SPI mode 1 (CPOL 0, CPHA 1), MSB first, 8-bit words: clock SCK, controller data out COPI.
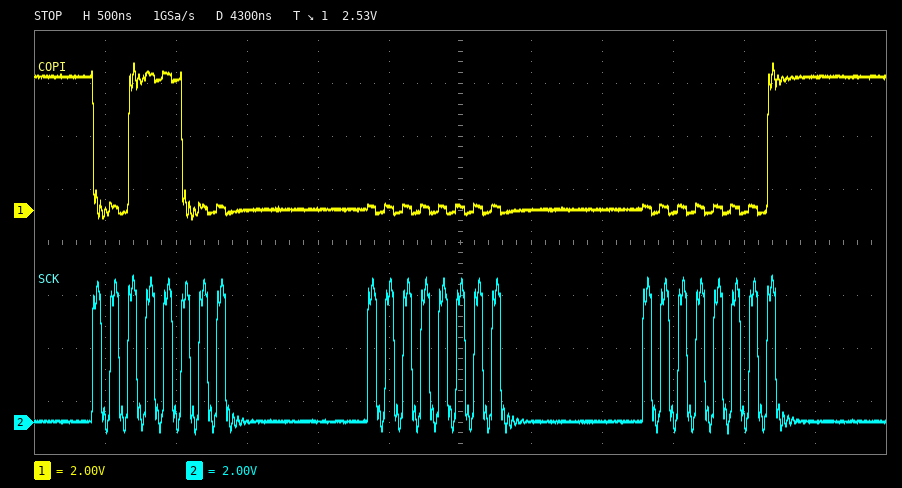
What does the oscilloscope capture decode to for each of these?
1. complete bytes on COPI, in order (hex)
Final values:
38 00 01
